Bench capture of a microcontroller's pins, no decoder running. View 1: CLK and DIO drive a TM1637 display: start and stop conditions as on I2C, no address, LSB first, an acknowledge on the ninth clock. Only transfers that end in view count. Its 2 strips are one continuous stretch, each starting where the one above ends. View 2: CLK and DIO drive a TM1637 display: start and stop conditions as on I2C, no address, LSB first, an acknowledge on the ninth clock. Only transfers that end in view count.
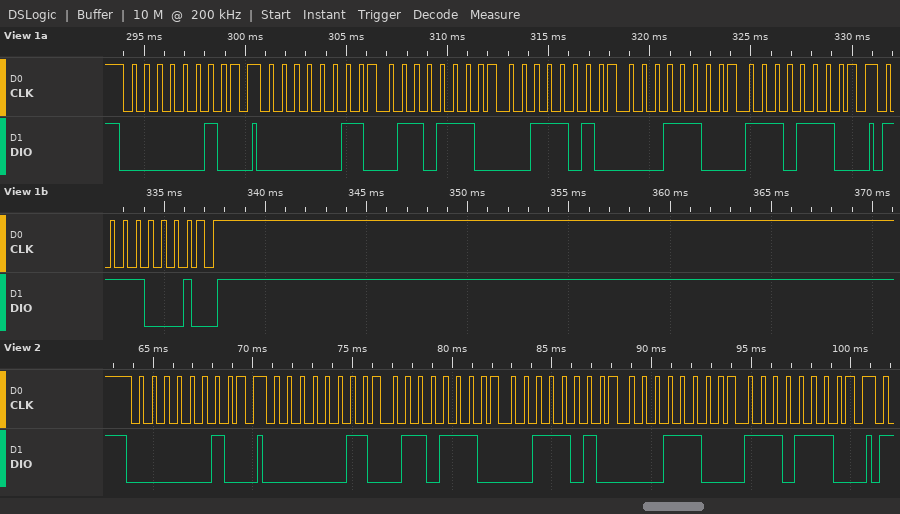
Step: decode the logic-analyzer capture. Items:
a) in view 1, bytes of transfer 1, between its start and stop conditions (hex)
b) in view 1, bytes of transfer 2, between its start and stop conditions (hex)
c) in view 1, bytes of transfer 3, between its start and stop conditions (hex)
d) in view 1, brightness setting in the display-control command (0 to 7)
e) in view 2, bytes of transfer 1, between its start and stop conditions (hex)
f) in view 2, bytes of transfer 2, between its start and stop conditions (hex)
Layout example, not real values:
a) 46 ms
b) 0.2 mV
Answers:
a) 40
b) C0 76 5C 38 77
c) 8F
d) 7
e) 40
f) C0 76 5C 38 77
